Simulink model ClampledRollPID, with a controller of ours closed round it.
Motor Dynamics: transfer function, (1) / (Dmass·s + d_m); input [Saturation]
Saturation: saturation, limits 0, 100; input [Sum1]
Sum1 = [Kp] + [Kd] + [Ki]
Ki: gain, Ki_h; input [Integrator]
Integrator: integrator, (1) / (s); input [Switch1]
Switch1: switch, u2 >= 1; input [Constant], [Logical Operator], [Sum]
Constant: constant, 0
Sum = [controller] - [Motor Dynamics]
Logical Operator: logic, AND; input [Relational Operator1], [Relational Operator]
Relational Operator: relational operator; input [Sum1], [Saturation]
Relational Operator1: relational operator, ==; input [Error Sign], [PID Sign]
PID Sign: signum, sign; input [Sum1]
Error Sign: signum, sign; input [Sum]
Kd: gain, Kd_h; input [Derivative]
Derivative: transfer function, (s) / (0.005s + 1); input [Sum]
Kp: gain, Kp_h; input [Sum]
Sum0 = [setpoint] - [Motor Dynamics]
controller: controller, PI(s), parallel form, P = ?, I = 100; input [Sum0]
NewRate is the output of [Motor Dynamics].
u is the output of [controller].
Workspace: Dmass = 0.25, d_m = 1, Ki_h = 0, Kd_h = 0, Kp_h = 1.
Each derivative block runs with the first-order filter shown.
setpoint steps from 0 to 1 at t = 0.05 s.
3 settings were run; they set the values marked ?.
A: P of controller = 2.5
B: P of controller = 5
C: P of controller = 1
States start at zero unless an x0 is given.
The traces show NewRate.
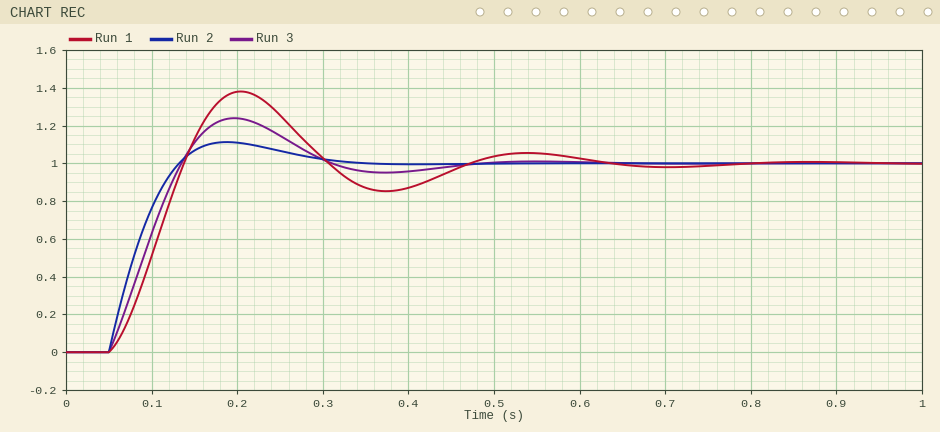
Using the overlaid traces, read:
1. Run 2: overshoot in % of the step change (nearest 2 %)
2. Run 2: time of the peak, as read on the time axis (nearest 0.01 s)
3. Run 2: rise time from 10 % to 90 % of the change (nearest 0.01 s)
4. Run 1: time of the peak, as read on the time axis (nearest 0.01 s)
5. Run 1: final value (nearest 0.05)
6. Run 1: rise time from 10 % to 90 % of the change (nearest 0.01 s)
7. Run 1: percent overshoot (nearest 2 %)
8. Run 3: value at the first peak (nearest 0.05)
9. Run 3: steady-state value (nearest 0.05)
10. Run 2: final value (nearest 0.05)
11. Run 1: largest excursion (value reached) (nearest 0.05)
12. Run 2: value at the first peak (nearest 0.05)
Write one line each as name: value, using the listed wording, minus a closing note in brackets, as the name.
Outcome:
Run 2: overshoot in % of the step change: 12 %
Run 2: time of the peak, as read on the time axis: 0.19 s
Run 2: rise time from 10 % to 90 % of the change: 0.06 s
Run 1: time of the peak, as read on the time axis: 0.20 s
Run 1: final value: 1.00
Run 1: rise time from 10 % to 90 % of the change: 0.06 s
Run 1: percent overshoot: 38 %
Run 3: value at the first peak: 1.25
Run 3: steady-state value: 1.00
Run 2: final value: 1.00
Run 1: largest excursion (value reached): 1.40
Run 2: value at the first peak: 1.10
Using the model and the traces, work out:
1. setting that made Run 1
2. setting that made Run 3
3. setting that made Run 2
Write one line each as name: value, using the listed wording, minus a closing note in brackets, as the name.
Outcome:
setting that made Run 1: C
setting that made Run 3: A
setting that made Run 2: B
